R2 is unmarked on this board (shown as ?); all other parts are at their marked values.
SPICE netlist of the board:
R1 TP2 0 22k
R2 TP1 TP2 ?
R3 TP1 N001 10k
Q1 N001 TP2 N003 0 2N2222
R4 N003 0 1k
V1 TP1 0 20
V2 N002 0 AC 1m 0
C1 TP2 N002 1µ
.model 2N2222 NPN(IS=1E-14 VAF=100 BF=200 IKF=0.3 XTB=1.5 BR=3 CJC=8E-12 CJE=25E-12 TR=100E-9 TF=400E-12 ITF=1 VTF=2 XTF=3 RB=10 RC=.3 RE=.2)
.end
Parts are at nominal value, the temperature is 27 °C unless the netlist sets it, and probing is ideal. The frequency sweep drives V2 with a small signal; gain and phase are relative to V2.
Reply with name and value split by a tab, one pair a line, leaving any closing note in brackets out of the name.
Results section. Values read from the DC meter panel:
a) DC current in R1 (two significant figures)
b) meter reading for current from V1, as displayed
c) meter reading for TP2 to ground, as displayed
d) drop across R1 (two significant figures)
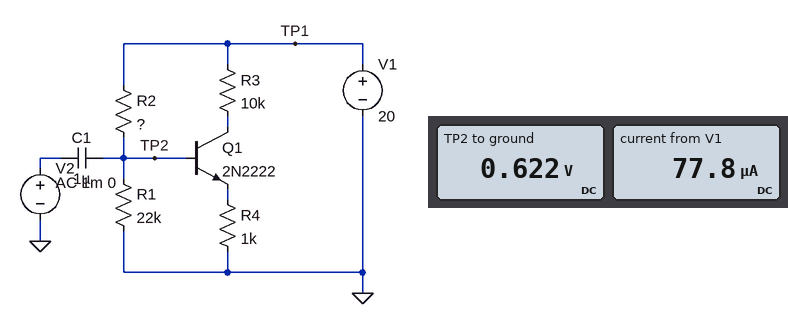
DC current in R1	28 µA
meter reading for current from V1, as displayed	77.8 µA
meter reading for TP2 to ground, as displayed	0.622 V
drop across R1	620 mV
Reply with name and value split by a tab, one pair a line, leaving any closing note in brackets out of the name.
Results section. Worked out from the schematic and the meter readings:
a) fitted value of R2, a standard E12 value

fitted value of R2, a standard E12 value	680 kΩ
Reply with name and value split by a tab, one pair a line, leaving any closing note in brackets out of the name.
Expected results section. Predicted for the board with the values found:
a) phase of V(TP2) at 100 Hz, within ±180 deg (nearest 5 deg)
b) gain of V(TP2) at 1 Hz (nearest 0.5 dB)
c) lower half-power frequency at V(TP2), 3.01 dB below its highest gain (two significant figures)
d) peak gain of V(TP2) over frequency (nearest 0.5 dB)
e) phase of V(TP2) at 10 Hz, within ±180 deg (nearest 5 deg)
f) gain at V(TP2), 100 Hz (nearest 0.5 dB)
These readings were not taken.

phase of V(TP2) at 100 Hz, within ±180 deg	5 deg
gain of V(TP2) at 1 Hz	-18.0 dB
lower half-power frequency at V(TP2), 3.01 dB below its highest gain	7.9 Hz
peak gain of V(TP2) over frequency	0 dB
phase of V(TP2) at 10 Hz, within ±180 deg	40 deg
gain at V(TP2), 100 Hz	0 dB
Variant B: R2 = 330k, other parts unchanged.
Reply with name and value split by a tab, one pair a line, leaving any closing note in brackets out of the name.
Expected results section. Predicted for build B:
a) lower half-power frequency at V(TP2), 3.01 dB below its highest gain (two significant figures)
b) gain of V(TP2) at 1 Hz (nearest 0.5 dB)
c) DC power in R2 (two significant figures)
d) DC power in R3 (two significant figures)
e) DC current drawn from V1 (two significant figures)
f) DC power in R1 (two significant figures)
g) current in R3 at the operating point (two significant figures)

lower half-power frequency at V(TP2), 3.01 dB below its highest gain	8.4 Hz
gain of V(TP2) at 1 Hz	-18.5 dB
DC power in R2	1.1 mW
DC power in R3	3.1 mW
DC current drawn from V1	620 µA
DC power in R1	65 µW
current in R3 at the operating point	560 µA
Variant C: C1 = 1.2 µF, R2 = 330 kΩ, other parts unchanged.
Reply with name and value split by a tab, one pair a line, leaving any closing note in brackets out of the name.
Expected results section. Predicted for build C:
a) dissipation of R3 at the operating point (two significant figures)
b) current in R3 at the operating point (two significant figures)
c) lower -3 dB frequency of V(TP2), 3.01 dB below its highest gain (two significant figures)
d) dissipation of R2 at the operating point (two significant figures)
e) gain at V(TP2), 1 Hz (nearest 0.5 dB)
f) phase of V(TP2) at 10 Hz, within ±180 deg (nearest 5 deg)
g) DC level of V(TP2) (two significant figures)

dissipation of R3 at the operating point	3.1 mW
current in R3 at the operating point	560 µA
lower -3 dB frequency of V(TP2), 3.01 dB below its highest gain	7.0 Hz
dissipation of R2 at the operating point	1.1 mW
gain at V(TP2), 1 Hz	-17.0 dB
phase of V(TP2) at 10 Hz, within ±180 deg	35 deg
DC level of V(TP2)	1.2 V
